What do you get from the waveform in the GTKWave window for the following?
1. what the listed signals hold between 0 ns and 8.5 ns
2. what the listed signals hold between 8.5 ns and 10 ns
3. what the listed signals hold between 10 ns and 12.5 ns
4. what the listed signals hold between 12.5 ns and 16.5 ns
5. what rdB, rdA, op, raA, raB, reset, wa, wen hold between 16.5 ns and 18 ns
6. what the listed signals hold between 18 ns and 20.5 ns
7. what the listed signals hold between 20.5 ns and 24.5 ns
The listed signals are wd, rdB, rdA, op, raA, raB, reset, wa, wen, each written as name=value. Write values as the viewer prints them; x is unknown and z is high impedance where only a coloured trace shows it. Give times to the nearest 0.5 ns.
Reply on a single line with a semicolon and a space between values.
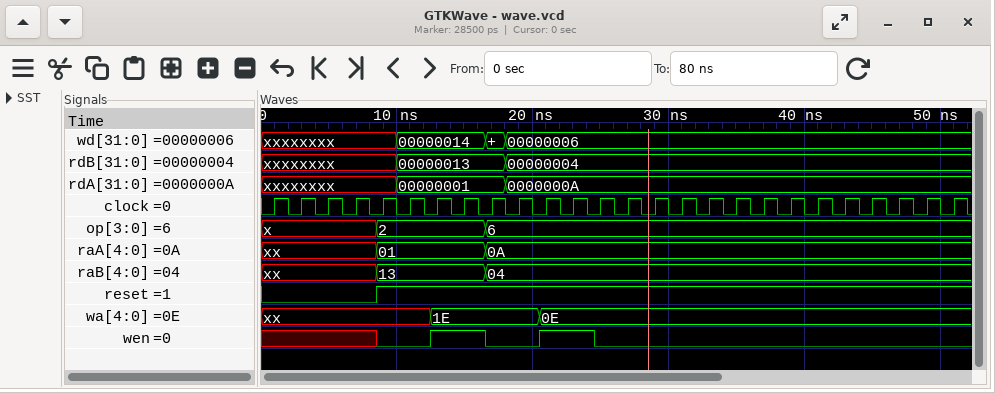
wd=xxxxxxxx, rdB=xxxxxxxx, rdA=xxxxxxxx, op=x, raA=xx, raB=xx, reset=0, wa=xx, wen=x; wd=xxxxxxxx, rdB=xxxxxxxx, rdA=xxxxxxxx, op=2, raA=01, raB=13, reset=1, wa=xx, wen=0; wd=00000014, rdB=00000013, rdA=00000001, op=2, raA=01, raB=13, reset=1, wa=xx, wen=0; wd=00000014, rdB=00000013, rdA=00000001, op=2, raA=01, raB=13, reset=1, wa=1E, wen=1; rdB=00000013, rdA=00000001, op=6, raA=0A, raB=04, reset=1, wa=1E, wen=0; wd=00000006, rdB=00000004, rdA=0000000A, op=6, raA=0A, raB=04, reset=1, wa=1E, wen=0; wd=00000006, rdB=00000004, rdA=0000000A, op=6, raA=0A, raB=04, reset=1, wa=0E, wen=1
